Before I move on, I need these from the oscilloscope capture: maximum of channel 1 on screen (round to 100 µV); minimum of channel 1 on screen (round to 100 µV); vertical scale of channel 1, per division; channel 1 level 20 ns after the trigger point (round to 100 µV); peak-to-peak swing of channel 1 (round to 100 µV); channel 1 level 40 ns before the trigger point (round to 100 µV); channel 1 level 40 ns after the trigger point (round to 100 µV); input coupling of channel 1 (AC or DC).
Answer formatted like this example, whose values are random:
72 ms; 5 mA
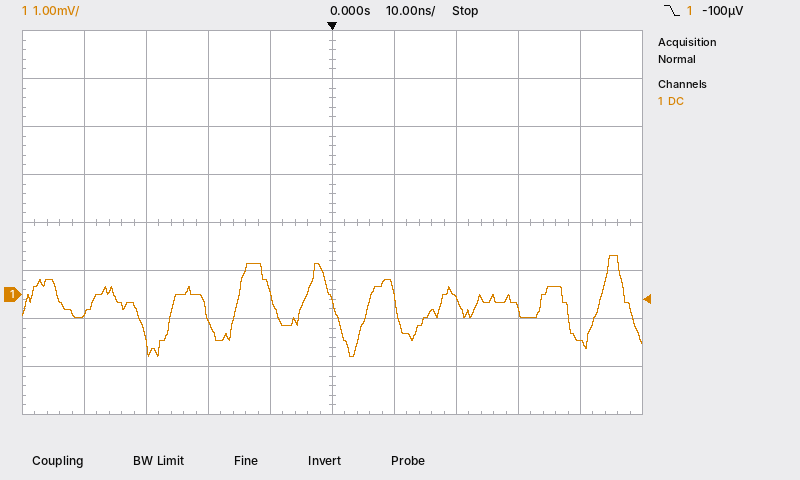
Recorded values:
800 µV; -1.3 mV; 1 mV; -100 µV; 2.1 mV; -400 µV; -1.0 mV; DC
